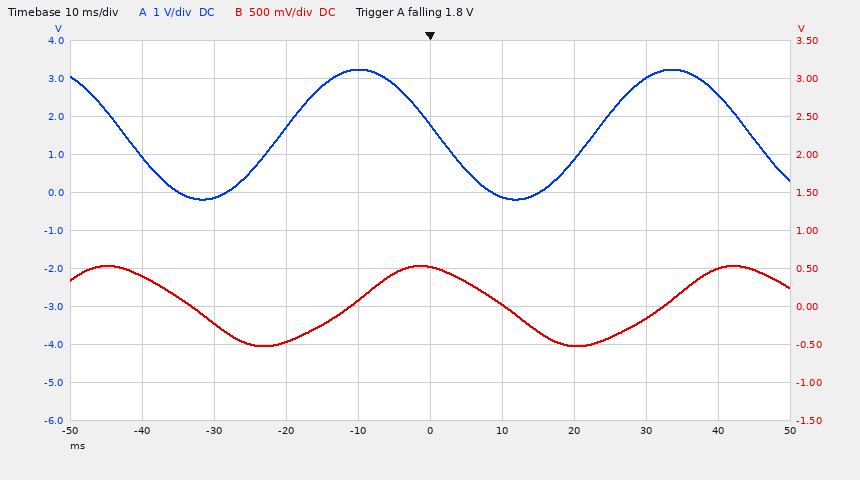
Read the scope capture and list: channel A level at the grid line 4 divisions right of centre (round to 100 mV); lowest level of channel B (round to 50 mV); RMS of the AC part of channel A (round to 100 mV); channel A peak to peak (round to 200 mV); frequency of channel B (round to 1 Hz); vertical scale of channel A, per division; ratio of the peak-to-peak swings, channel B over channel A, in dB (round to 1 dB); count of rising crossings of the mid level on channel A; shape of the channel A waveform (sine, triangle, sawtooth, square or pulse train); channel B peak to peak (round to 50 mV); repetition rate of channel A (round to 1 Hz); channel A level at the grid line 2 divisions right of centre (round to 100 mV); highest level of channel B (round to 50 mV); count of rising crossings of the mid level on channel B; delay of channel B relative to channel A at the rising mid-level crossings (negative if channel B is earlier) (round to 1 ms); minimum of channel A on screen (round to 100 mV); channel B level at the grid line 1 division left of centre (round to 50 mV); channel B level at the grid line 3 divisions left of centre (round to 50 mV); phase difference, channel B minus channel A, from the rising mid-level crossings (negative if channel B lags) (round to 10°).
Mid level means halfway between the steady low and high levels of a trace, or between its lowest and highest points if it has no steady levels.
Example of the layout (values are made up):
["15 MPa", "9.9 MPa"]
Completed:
["2.6 V", "-500 mV", "1.2 V", "3.4 V", "23 Hz", "1 V", "-10 dB", "2", "sine", "1.05 V", "23 Hz", "900 mV", "550 mV", "2", "+10 ms", "-200 mV", "100 mV", "-200 mV", "-80°"]
